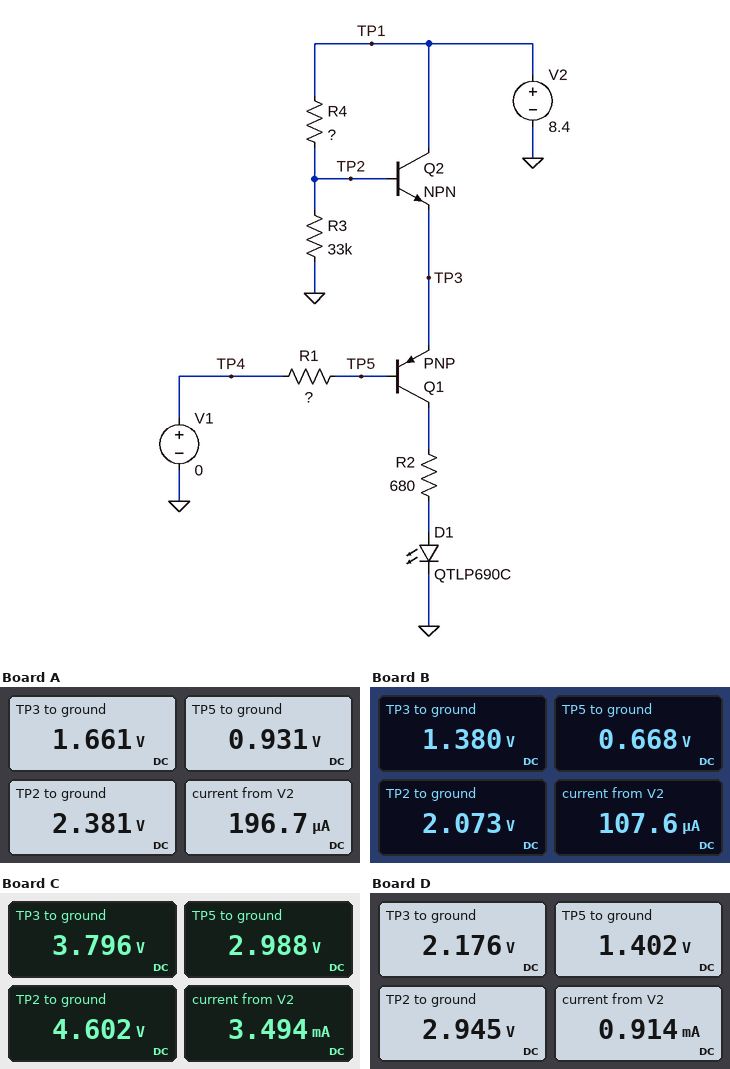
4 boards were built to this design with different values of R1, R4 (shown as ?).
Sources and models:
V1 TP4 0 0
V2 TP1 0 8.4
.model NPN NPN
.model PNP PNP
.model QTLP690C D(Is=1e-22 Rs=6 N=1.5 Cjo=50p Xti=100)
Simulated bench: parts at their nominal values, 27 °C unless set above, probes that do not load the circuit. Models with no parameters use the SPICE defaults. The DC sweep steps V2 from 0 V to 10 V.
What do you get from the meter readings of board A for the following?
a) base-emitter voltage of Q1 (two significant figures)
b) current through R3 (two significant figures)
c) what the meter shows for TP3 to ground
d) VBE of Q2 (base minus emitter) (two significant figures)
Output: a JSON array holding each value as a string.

["-730 mV", "72 µA", "1.661 V", "720 mV"]
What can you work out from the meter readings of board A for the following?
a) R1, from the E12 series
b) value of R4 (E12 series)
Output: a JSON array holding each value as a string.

["15 kΩ", "82 kΩ"]
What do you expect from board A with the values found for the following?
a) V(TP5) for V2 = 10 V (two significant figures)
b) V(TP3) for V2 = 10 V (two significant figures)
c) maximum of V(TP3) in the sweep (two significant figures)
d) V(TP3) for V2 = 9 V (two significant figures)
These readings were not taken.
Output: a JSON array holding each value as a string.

["1.2 V", "2.0 V", "2.0 V", "1.8 V"]
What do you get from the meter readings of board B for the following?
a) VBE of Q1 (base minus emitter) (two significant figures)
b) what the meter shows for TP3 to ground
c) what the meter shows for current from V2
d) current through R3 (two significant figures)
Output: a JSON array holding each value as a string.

["-710 mV", "1.380 V", "107.6 µA", "63 µA"]
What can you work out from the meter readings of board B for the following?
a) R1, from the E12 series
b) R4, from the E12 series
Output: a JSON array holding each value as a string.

["15 kΩ", "100 kΩ"]
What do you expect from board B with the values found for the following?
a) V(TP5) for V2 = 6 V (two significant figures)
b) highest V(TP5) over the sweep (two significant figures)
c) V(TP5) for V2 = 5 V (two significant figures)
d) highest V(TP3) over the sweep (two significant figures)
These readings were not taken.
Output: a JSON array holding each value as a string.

["160 mV", "980 mV", "19 mV", "1.7 V"]
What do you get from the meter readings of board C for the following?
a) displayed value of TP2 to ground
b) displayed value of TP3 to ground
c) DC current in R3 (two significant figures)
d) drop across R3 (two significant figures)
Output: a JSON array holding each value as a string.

["4.602 V", "3.796 V", "140 µA", "4.6 V"]
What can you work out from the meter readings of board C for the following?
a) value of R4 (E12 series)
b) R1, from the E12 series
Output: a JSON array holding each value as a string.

["22 kΩ", "6.8 kΩ"]
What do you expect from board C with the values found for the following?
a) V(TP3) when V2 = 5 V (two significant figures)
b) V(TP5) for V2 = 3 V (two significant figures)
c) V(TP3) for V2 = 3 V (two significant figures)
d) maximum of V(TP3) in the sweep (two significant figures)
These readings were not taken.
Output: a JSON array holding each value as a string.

["2.1 V", "380 mV", "1.1 V", "4.6 V"]
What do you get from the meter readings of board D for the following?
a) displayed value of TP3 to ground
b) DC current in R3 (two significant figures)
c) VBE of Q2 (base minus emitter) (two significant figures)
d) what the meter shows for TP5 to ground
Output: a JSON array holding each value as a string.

["2.176 V", "89 µA", "770 mV", "1.402 V"]
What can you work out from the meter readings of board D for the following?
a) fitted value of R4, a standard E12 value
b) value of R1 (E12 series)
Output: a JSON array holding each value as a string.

["56 kΩ", "8.2 kΩ"]
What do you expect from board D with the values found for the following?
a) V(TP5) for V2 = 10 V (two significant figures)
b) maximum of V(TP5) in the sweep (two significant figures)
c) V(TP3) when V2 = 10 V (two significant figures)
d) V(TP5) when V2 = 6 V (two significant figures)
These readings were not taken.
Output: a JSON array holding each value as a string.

["1.8 V", "1.8 V", "2.6 V", "760 mV"]
